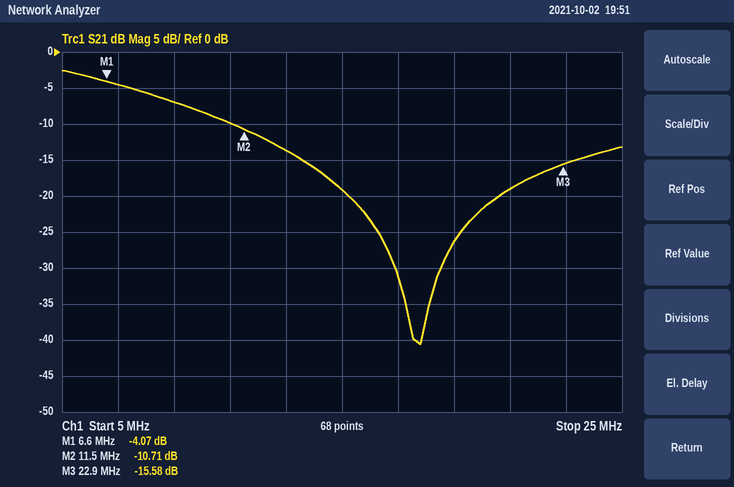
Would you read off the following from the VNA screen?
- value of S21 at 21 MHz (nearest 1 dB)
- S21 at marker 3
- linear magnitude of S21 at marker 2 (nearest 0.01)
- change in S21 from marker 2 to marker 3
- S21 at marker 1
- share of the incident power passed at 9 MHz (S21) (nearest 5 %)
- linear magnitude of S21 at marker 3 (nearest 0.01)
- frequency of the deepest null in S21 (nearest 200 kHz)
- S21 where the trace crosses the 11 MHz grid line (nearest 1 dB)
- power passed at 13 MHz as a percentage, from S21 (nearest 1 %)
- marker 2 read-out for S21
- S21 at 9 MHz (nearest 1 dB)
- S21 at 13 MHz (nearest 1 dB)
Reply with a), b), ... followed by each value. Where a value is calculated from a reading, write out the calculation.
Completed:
a) -19 dB
b) -15.58 dB
c) 10^(-10.71/20) ≈ 0.29
d) -15.58 − (-10.71) = -4.87 dB
e) -4.07 dB
f) 10^(-7/10) ≈ 20 %
g) 10^(-15.58/20) ≈ 0.17
h) 17.8 MHz
i) -10 dB
j) 10^(-14/10) ≈ 4 %
k) -10.71 dB
l) -7 dB
m) -14 dB
